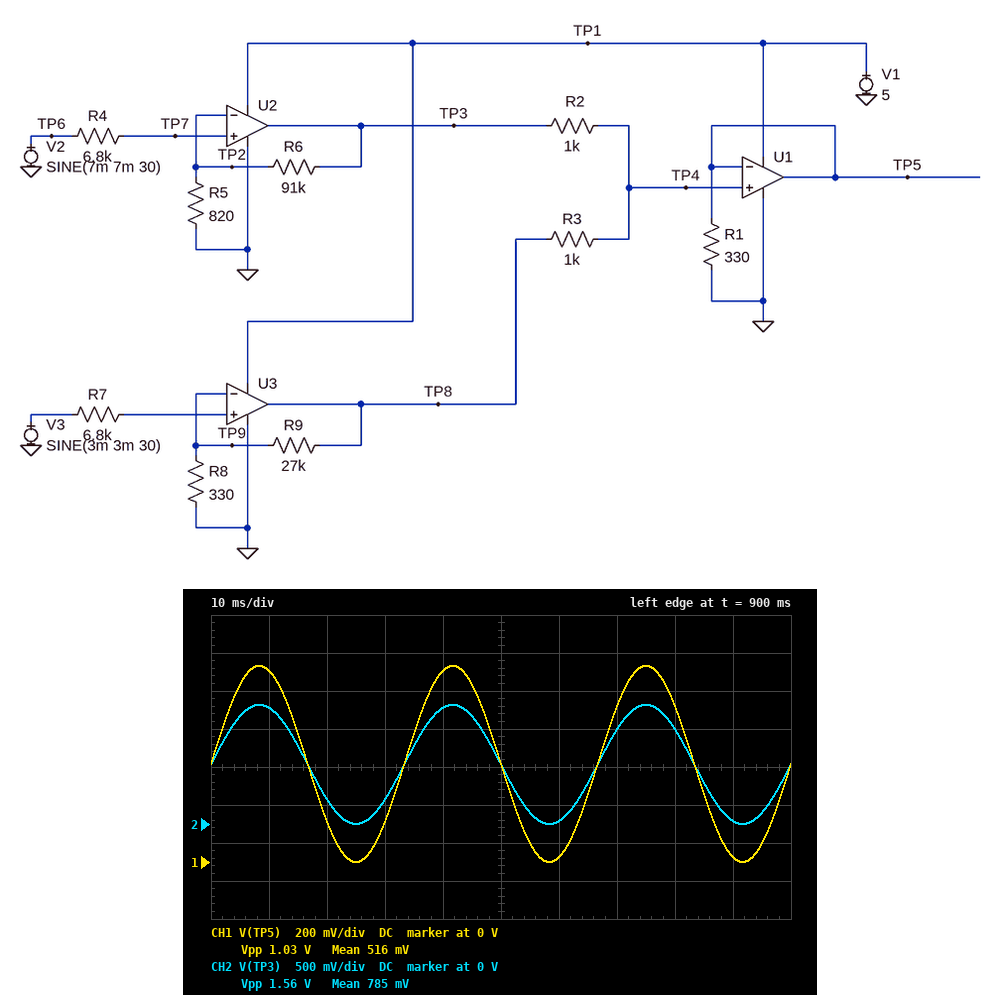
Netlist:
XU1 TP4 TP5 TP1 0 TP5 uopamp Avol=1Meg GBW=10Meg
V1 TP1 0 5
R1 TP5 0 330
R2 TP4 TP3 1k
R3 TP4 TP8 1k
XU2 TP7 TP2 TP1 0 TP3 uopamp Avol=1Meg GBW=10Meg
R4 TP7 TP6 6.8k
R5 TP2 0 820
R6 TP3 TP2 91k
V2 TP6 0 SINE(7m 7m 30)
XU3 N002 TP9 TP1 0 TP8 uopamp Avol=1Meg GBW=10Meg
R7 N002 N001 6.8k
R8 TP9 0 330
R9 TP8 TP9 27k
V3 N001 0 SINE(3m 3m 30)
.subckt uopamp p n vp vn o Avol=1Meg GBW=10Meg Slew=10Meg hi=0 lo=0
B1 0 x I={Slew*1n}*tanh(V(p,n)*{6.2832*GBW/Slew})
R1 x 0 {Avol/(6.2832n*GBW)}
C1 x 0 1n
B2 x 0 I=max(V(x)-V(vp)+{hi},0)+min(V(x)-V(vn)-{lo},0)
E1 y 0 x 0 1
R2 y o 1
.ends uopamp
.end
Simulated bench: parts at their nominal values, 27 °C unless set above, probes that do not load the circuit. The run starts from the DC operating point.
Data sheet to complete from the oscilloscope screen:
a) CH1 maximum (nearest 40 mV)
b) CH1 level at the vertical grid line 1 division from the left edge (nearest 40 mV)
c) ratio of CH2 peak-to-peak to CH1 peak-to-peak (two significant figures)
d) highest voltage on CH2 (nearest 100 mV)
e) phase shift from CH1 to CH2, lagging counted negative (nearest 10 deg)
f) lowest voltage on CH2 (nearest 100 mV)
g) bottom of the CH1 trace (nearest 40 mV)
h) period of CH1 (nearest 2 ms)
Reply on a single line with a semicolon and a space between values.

1.04 V; 1.00 V; 1.5; 1.6 V; 0 deg; 0 V; 0 V; 34 ms
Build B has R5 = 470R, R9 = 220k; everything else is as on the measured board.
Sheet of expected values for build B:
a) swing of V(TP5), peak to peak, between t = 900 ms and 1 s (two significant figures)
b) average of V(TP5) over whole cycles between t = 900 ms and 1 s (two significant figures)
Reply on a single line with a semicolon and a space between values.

3.4 V; 1.7 V
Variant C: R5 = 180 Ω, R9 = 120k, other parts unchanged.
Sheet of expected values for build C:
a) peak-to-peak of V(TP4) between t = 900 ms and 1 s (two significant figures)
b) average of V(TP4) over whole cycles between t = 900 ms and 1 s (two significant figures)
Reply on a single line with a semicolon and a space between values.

3.6 V; 2.1 V
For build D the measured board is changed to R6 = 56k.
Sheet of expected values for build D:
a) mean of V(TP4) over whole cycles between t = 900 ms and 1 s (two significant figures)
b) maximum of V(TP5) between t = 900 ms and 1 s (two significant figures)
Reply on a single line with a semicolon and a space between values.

370 mV; 730 mV
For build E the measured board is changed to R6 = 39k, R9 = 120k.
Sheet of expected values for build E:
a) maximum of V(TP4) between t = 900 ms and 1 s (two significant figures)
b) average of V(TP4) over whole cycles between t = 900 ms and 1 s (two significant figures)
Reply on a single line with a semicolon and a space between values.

1.4 V; 720 mV
